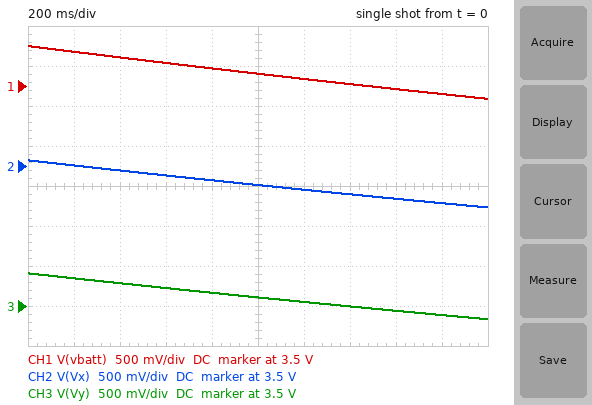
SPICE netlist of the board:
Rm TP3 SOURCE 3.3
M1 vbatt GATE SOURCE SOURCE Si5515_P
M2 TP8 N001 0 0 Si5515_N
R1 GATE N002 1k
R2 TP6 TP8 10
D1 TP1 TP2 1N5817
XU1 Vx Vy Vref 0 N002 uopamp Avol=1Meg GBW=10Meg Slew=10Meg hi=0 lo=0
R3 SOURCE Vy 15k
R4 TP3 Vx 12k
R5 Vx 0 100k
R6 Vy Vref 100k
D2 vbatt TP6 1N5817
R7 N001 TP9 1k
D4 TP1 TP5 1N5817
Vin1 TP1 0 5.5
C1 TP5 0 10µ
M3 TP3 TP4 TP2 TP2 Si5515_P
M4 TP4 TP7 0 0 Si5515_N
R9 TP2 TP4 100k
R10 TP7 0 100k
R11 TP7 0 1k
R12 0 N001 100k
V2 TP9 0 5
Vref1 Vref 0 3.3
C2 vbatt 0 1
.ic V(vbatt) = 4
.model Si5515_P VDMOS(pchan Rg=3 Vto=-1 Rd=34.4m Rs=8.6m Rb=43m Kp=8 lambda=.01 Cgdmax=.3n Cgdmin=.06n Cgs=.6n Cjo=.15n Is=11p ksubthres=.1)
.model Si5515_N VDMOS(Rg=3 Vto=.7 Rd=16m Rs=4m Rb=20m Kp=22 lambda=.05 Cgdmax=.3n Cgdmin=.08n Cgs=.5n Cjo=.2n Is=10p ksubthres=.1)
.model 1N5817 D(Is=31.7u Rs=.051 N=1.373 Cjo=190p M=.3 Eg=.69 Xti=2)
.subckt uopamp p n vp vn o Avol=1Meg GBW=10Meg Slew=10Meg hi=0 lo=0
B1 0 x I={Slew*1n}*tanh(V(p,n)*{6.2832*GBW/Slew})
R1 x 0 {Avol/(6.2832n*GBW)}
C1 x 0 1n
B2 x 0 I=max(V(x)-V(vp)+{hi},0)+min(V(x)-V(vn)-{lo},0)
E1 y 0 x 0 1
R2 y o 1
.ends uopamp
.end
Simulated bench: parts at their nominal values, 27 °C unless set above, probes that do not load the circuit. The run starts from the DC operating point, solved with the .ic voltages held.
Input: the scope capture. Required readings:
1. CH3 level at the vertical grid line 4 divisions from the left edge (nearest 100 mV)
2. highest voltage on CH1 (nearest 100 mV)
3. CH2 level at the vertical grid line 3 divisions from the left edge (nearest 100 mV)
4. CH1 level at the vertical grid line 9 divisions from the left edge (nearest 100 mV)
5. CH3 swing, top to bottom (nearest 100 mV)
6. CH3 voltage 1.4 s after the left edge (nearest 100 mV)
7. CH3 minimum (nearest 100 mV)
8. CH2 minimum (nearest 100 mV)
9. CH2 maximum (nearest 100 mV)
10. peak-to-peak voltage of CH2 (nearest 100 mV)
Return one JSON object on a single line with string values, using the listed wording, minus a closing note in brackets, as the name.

{"CH3 level at the vertical grid line 4 divisions from the left edge": "3.7 V", "highest voltage on CH1": "4.0 V", "CH2 level at the vertical grid line 3 divisions from the left edge": "3.4 V", "CH1 level at the vertical grid line 9 divisions from the left edge": "3.4 V", "CH3 swing, top to bottom": "600 mV", "CH3 voltage 1.4 s after the left edge": "3.5 V", "CH3 minimum": "3.3 V", "CH2 minimum": "3.0 V", "CH2 maximum": "3.6 V", "peak-to-peak voltage of CH2": "600 mV"}
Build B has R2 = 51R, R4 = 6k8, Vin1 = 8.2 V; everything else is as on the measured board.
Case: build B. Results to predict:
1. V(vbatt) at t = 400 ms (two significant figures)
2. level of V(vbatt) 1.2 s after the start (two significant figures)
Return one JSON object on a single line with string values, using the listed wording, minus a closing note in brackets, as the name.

{"V(vbatt) at t = 400 ms": "4.0 V", "level of V(vbatt) 1.2 s after the start": "3.9 V"}
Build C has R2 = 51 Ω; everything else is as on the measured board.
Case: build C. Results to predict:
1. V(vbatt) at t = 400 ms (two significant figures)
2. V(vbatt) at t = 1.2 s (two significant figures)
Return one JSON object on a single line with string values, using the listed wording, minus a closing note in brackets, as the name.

{"V(vbatt) at t = 400 ms": "4.0 V", "V(vbatt) at t = 1.2 s": "3.9 V"}
